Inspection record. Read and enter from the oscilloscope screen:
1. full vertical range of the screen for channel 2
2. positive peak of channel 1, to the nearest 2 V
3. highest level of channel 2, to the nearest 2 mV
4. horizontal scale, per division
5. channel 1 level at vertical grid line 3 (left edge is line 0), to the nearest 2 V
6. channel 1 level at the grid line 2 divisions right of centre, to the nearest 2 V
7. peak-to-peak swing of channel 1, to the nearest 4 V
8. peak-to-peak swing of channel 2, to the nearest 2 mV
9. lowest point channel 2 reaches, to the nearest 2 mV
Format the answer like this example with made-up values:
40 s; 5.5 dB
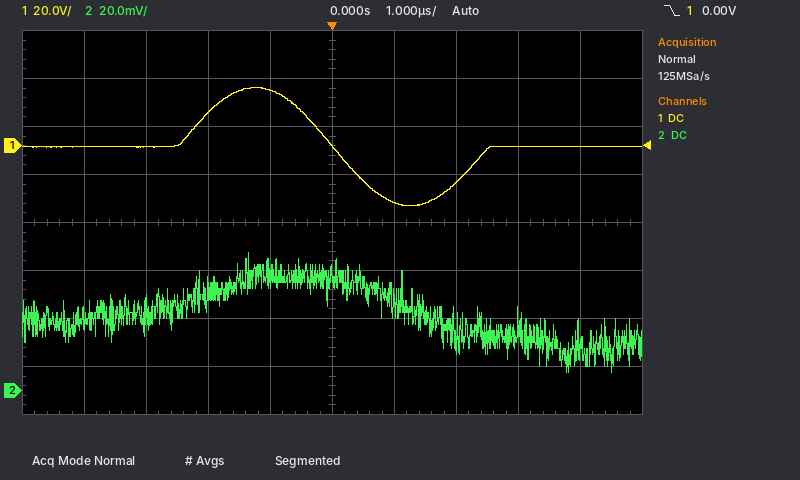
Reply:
160 mV; 24 V; 58 mV; 1 µs; 14 V; -16 V; 48 V; 50 mV; 8 mV
